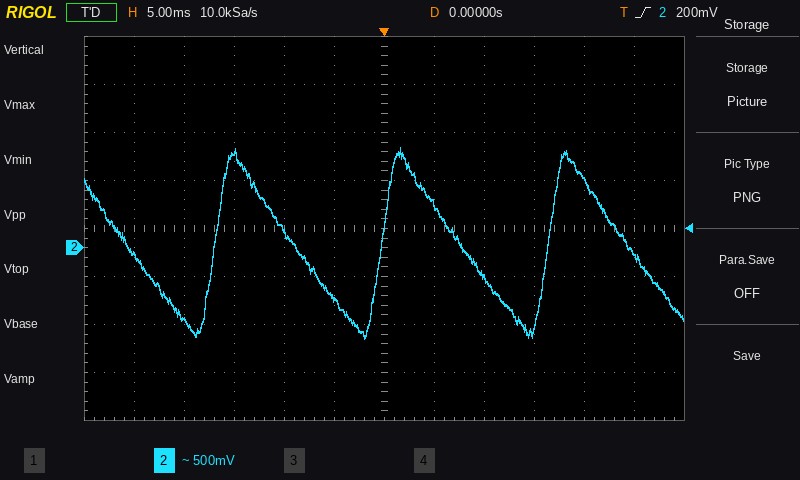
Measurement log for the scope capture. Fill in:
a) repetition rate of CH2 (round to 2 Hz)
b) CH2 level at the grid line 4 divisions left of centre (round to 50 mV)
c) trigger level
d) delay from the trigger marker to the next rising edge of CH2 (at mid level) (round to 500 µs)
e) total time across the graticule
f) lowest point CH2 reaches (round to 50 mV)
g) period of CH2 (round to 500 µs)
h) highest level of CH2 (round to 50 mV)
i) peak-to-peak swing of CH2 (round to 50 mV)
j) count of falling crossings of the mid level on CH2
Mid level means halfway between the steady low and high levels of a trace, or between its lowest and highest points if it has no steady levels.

60 Hz
-750 mV
200 mV
16.5 ms
60 ms
-950 mV
16.5 ms
1.05 V
2.00 V
4
